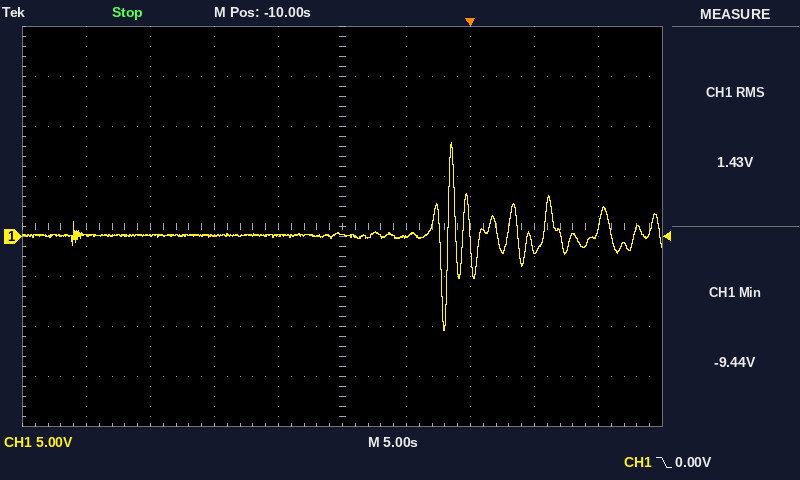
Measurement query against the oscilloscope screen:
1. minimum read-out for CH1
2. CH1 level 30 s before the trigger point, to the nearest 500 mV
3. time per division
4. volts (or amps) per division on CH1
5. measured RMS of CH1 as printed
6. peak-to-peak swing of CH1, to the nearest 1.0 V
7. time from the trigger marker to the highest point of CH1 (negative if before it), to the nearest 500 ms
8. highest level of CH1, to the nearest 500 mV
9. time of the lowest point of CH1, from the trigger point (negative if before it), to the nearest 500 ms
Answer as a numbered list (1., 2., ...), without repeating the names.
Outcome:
1. -9.44 V
2. 0.0 V
3. 5 s
4. 5 V
5. 1.43 V
6. 19.0 V
7. -1.5 s
8. 9.5 V
9. -2.0 s
